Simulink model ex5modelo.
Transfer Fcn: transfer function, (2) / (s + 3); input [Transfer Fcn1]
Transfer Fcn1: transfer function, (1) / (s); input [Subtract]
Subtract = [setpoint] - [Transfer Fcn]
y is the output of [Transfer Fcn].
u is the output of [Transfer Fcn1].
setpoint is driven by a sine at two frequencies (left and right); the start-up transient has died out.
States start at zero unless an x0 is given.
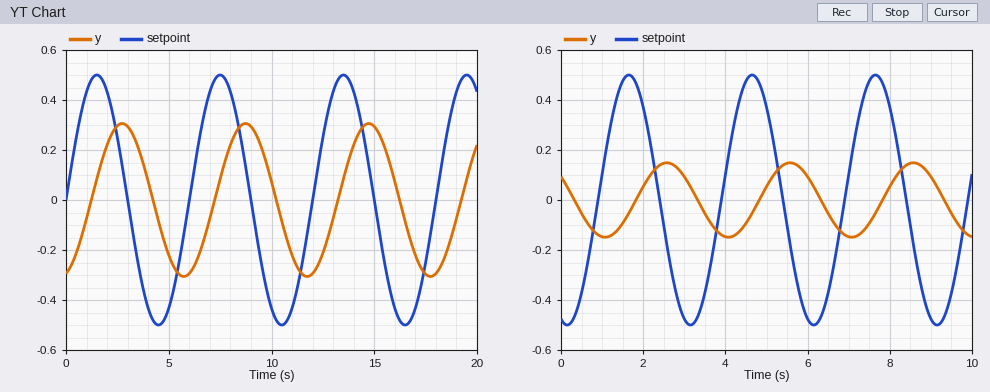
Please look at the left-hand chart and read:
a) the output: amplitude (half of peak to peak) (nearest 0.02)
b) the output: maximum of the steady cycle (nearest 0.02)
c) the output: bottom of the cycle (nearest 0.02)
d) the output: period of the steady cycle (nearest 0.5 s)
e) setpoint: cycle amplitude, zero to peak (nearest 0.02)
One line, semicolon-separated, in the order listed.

0.30; 0.30; -0.30; 6.0 s; 0.50
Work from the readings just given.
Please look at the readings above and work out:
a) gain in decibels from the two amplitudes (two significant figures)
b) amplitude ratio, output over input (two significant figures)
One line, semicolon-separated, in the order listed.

-4.4 dB; 0.60
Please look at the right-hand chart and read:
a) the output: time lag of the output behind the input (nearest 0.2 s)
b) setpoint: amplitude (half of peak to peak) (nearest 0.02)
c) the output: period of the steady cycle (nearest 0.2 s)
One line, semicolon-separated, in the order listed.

1.0 s; 0.50; 3.0 s
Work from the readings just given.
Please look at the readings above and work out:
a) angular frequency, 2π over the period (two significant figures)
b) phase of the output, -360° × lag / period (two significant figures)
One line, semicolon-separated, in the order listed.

2.1 rad/s; -120°
